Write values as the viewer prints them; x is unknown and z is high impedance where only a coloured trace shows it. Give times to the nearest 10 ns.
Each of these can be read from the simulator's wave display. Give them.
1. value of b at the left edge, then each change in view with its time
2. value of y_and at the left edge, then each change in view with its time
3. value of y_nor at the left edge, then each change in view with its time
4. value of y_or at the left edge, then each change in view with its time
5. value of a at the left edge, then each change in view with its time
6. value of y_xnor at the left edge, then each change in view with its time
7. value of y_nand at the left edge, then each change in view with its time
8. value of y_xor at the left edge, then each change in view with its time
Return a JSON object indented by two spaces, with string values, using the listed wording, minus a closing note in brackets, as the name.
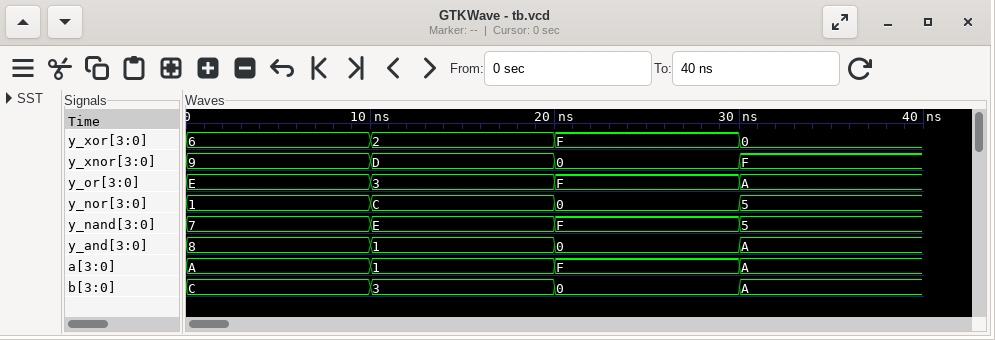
{
  "value of b at the left edge, then each change in view with its time": "C, 3 at 10 ns, 0 at 20 ns, A at 30 ns",
  "value of y_and at the left edge, then each change in view with its time": "8, 1 at 10 ns, 0 at 20 ns, A at 30 ns",
  "value of y_nor at the left edge, then each change in view with its time": "1, C at 10 ns, 0 at 20 ns, 5 at 30 ns",
  "value of y_or at the left edge, then each change in view with its time": "E, 3 at 10 ns, F at 20 ns, A at 30 ns",
  "value of a at the left edge, then each change in view with its time": "A, 1 at 10 ns, F at 20 ns, A at 30 ns",
  "value of y_xnor at the left edge, then each change in view with its time": "9, D at 10 ns, 0 at 20 ns, F at 30 ns",
  "value of y_nand at the left edge, then each change in view with its time": "7, E at 10 ns, F at 20 ns, 5 at 30 ns",
  "value of y_xor at the left edge, then each change in view with its time": "6, 2 at 10 ns, F at 20 ns, 0 at 30 ns"
}
